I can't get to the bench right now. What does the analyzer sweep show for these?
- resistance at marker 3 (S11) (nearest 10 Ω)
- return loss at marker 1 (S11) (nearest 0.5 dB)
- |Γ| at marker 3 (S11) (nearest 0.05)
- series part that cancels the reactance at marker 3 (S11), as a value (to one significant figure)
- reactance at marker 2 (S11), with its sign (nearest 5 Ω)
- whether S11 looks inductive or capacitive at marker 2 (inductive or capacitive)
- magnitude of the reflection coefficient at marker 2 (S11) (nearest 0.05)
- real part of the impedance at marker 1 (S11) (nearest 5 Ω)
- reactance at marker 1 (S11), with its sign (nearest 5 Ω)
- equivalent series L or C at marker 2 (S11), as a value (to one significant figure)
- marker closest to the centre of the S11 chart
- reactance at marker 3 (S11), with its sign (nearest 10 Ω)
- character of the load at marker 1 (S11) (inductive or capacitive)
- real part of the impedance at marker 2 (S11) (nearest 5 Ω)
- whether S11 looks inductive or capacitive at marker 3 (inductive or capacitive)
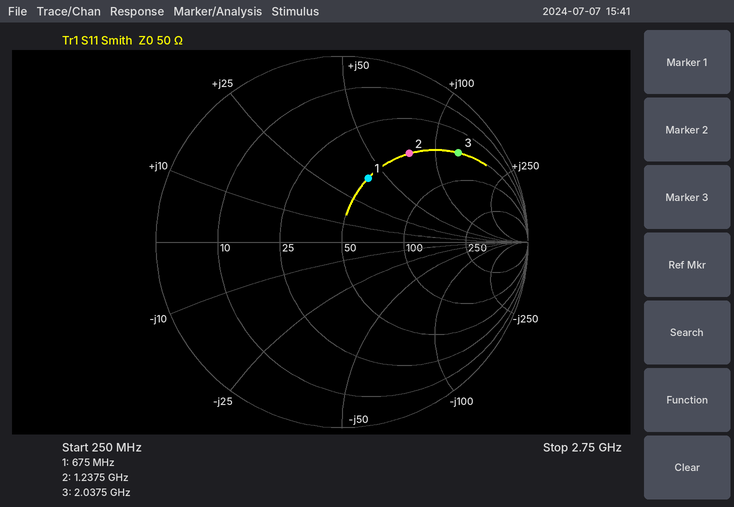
50 Ω
8.5 dB
0.80
600 fF
+75 Ω
inductive
0.60
50 Ω
+40 Ω
10 nH
marker 1
+130 Ω
inductive
50 Ω
inductive
